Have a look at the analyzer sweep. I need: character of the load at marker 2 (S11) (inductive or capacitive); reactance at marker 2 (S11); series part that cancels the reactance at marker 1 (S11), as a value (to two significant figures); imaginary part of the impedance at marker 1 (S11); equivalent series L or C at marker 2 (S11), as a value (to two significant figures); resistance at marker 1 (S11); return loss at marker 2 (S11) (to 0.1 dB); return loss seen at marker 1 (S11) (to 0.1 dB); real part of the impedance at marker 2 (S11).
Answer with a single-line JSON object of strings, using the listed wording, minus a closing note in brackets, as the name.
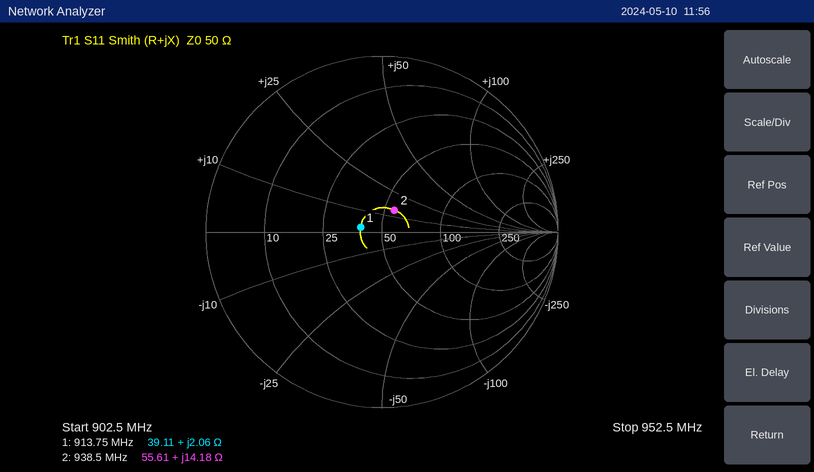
{"character of the load at marker 2 (S11)": "inductive", "reactance at marker 2": "+14.18 Ω", "series part that cancels the reactance at marker 1 (S11), as a value": "85 pF", "imaginary part of the impedance at marker 1": "+2.06 Ω", "equivalent series L or C at marker 2 (S11), as a value": "2.4 nH", "resistance at marker 1": "39.11 Ω", "return loss at marker 2 (S11)": "16.9 dB", "return loss seen at marker 1 (S11)": "18.1 dB", "real part of the impedance at marker 2": "55.61 Ω"}
